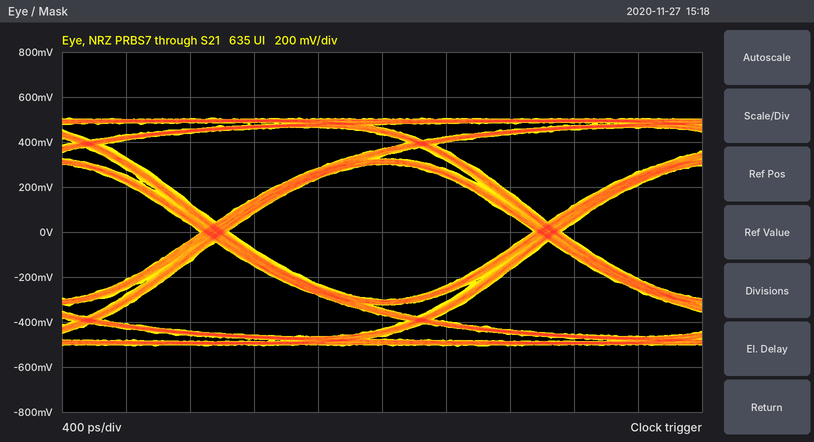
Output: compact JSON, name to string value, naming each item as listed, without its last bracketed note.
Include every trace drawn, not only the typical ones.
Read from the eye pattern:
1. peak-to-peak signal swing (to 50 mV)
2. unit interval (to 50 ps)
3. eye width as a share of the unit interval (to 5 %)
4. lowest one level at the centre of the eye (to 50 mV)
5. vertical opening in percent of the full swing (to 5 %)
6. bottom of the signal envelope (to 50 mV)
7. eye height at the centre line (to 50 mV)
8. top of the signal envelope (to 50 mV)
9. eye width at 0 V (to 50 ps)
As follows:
{"peak-to-peak signal swing": "1.00 V", "unit interval": "2.10 ns", "eye width as a share of the unit interval": "90 %", "lowest one level at the centre of the eye": "300 mV", "vertical opening in percent of the full swing": "60 %", "bottom of the signal envelope": "-500 mV", "eye height at the centre line": "600 mV", "top of the signal envelope": "500 mV", "eye width at 0 V": "1.90 ns"}
